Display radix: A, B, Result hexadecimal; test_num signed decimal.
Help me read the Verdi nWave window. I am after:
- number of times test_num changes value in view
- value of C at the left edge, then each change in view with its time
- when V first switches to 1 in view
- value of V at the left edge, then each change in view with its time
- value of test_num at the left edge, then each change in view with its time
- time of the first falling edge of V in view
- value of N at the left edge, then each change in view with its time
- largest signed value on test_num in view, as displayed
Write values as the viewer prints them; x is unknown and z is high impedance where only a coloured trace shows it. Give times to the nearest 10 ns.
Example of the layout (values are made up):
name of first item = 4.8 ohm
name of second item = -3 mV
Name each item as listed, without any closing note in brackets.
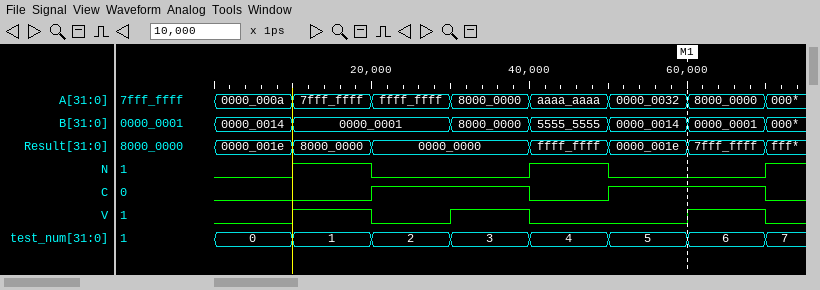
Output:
number of times test_num changes value in view = 7
value of C at the left edge, then each change in view with its time = 0, 1 at 20 ns, 0 at 40 ns, 1 at 50 ns, 0 at 70 ns
when V first switches to 1 in view = 10 ns
value of V at the left edge, then each change in view with its time = 0, 1 at 10 ns, 0 at 20 ns, 1 at 30 ns, 0 at 40 ns, 1 at 60 ns, 0 at 70 ns
value of test_num at the left edge, then each change in view with its time = 0, 1 at 10 ns, 2 at 20 ns, 3 at 30 ns, 4 at 40 ns, 5 at 50 ns, 6 at 60 ns, 7 at 70 ns
time of the first falling edge of V in view = 20 ns
value of N at the left edge, then each change in view with its time = 0, 1 at 10 ns, 0 at 20 ns, 1 at 40 ns, 0 at 50 ns, 1 at 70 ns
largest signed value on test_num in view, as displayed = 7
